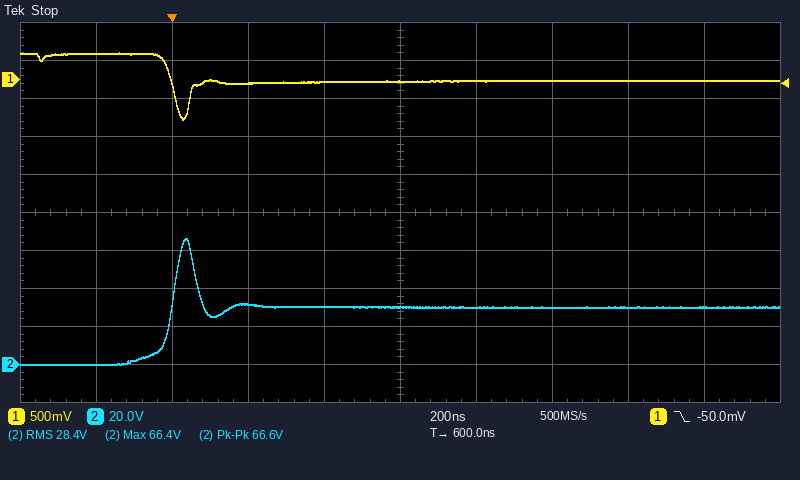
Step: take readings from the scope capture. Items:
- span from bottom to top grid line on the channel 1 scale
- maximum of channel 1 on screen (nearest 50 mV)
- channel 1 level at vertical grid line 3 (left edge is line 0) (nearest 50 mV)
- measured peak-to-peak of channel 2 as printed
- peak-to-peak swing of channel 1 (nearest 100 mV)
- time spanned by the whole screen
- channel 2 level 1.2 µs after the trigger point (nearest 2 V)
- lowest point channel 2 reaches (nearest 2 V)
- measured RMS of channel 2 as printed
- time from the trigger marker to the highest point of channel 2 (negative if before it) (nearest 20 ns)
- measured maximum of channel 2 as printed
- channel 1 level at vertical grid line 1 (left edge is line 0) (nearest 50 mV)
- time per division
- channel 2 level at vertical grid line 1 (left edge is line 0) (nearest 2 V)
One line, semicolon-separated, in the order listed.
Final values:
5 V; 350 mV; -50 mV; 66.6 V; 900 mV; 2 µs; 30 V; 0 V; 28.4 V; +40 ns; 66.4 V; 350 mV; 200 ns; 0 V
